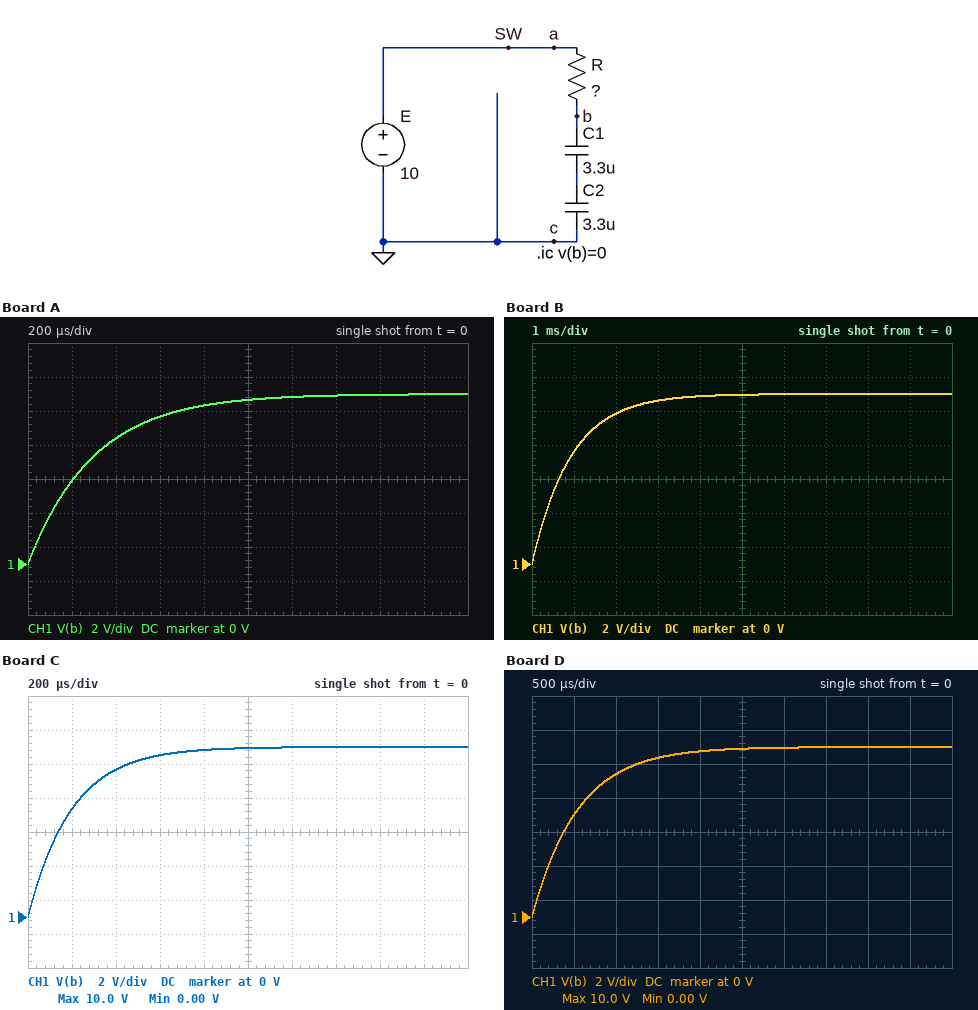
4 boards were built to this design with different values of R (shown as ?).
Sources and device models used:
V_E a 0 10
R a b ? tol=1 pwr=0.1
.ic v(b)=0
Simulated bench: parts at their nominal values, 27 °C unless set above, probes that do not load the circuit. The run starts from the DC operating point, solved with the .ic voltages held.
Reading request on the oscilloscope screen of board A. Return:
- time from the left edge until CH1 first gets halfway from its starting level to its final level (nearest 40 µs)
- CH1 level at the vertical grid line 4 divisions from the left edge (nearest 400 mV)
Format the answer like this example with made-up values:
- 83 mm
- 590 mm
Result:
- 200 µs
- 9.2 V
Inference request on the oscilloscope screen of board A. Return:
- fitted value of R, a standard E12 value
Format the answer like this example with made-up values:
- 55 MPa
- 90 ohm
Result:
- 180 Ω
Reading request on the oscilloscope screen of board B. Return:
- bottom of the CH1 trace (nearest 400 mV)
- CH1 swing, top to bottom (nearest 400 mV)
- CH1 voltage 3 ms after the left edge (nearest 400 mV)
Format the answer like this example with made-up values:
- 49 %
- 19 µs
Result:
- 0 V
- 10.0 V
- 9.6 V
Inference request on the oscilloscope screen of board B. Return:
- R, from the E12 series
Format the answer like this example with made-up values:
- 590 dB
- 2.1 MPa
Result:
- 560 Ω
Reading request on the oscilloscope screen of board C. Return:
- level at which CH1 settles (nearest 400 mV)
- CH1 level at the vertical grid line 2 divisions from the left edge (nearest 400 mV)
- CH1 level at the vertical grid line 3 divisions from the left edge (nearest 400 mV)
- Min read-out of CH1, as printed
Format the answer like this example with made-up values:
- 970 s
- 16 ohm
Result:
- 10.0 V
- 8.8 V
- 9.6 V
- 0.00 V
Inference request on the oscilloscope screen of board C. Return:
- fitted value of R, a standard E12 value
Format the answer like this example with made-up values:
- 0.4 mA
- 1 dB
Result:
- 120 Ω
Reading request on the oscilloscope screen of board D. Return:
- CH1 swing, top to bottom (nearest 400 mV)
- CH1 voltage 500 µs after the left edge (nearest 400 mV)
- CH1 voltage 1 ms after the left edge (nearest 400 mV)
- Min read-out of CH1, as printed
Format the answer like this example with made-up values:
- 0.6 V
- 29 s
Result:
- 10.0 V
- 6.0 V
- 8.4 V
- 0.00 V
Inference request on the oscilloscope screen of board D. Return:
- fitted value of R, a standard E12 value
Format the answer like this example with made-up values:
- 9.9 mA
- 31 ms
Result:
- 330 Ω
